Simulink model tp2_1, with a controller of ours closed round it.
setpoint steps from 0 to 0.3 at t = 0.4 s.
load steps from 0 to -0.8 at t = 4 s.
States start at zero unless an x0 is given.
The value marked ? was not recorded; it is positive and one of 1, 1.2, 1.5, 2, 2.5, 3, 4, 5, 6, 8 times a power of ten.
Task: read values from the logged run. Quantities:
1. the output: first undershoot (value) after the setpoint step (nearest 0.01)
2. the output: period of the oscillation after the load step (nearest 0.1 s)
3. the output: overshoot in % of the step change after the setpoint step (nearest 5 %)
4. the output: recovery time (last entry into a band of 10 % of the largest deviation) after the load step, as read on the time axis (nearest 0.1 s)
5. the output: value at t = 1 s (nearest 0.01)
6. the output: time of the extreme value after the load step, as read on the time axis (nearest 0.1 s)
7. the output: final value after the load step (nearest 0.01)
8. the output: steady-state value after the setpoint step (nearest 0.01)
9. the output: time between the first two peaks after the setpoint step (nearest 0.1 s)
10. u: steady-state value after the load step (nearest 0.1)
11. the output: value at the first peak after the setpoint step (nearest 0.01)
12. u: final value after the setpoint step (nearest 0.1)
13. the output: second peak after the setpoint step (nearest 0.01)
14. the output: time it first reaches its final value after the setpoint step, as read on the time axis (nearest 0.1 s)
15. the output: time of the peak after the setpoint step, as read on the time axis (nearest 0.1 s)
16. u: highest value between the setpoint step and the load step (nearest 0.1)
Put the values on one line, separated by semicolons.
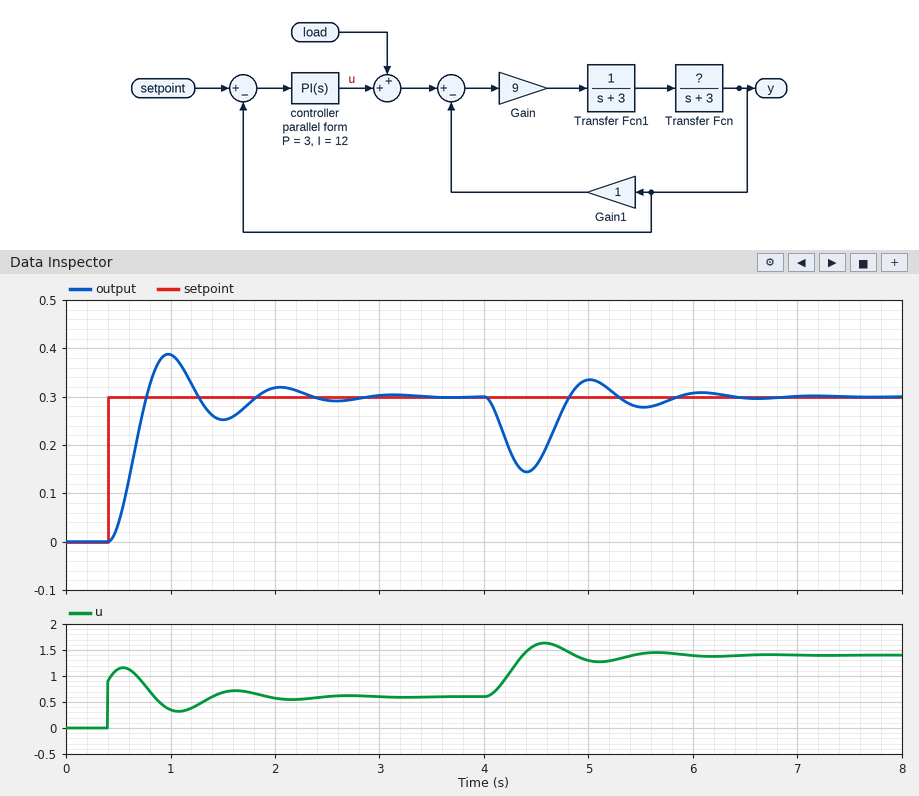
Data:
0.25; 1.1 s; 30 %; 5.7 s; 0.39; 4.4 s; 0.30; 0.30; 1.1 s; 1.4; 0.39; 0.6; 0.32; 0.8 s; 1.0 s; 1.2
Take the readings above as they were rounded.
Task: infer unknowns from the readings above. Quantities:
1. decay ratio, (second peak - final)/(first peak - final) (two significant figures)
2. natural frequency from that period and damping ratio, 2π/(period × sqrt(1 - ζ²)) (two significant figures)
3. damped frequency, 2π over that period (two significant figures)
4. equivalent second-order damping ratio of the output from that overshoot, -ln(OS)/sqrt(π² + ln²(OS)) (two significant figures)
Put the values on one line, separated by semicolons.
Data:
0.22; 6.1 rad/s; 5.7 rad/s; 0.36
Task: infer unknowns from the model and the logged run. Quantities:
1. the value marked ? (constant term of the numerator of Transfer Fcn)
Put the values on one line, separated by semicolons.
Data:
1
